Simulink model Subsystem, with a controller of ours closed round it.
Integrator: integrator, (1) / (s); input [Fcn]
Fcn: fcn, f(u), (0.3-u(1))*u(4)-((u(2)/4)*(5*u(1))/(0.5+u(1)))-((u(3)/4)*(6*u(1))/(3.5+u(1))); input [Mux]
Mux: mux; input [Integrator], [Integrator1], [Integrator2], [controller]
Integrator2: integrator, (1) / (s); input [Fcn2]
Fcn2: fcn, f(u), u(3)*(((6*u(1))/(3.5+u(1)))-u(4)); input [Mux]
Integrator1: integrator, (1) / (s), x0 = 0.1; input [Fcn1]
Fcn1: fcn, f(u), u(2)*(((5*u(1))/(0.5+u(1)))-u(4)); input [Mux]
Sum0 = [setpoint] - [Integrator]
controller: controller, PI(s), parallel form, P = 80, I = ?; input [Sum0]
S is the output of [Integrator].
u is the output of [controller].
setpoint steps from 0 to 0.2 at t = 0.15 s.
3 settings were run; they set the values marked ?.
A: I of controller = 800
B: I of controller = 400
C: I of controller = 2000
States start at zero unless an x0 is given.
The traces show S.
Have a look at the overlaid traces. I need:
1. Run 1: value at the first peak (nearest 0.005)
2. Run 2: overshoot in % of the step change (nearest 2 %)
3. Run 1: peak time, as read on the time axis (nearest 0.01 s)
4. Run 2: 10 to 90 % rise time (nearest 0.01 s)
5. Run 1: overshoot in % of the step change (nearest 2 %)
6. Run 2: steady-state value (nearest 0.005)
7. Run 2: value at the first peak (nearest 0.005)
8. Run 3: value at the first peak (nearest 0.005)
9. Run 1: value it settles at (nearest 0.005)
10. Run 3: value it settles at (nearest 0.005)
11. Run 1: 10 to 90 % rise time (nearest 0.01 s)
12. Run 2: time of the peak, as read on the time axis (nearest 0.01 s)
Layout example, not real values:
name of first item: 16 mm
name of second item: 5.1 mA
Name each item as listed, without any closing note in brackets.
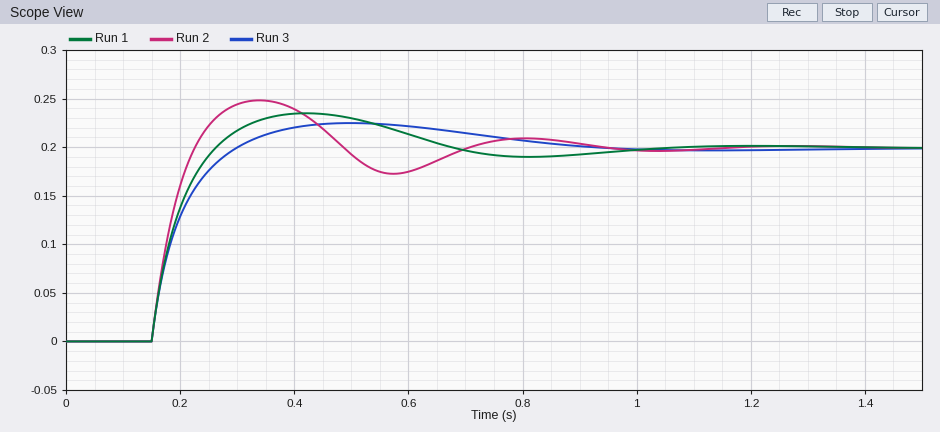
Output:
Run 1: value at the first peak: 0.235
Run 2: overshoot in % of the step change: 24 %
Run 1: peak time, as read on the time axis: 0.42 s
Run 2: 10 to 90 % rise time: 0.06 s
Run 1: overshoot in % of the step change: 18 %
Run 2: steady-state value: 0.200
Run 2: value at the first peak: 0.250
Run 3: value at the first peak: 0.225
Run 1: value it settles at: 0.200
Run 3: value it settles at: 0.200
Run 1: 10 to 90 % rise time: 0.08 s
Run 2: time of the peak, as read on the time axis: 0.34 s
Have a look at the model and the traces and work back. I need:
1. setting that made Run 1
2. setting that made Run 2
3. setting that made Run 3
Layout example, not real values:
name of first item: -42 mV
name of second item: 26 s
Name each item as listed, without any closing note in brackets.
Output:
setting that made Run 1: A
setting that made Run 2: C
setting that made Run 3: B
